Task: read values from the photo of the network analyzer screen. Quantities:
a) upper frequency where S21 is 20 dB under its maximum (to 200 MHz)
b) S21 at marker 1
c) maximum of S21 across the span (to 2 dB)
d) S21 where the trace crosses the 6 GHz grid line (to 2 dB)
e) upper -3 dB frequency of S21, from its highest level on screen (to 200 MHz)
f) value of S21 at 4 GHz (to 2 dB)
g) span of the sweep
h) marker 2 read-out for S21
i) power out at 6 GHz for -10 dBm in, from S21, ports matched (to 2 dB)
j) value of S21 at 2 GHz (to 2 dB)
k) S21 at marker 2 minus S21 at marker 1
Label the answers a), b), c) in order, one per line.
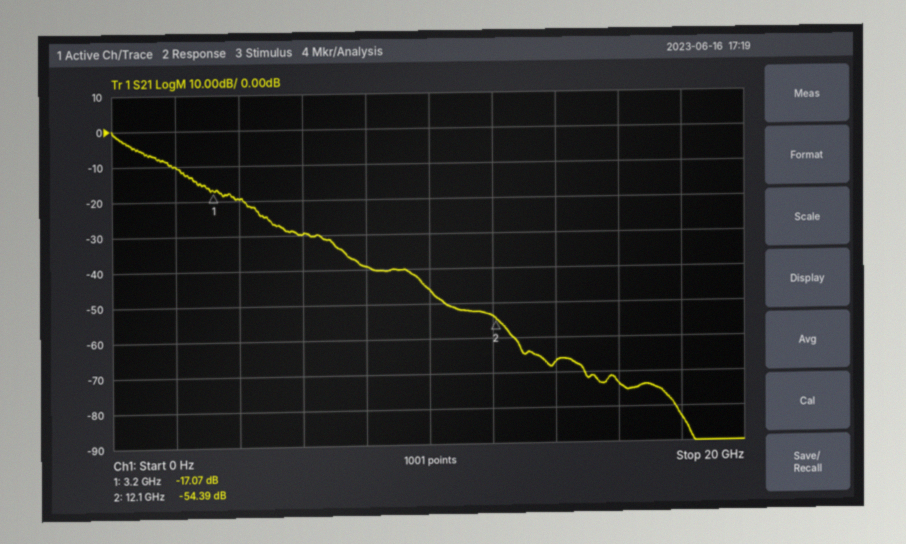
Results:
a) 4.2 GHz
b) -17.07 dB
c) 0 dB
d) -30 dB
e) 400 MHz
f) -20 dB
g) 20 GHz
h) -54.39 dB
i) -40 dBm
j) -10 dB
k) -37.32 dB
